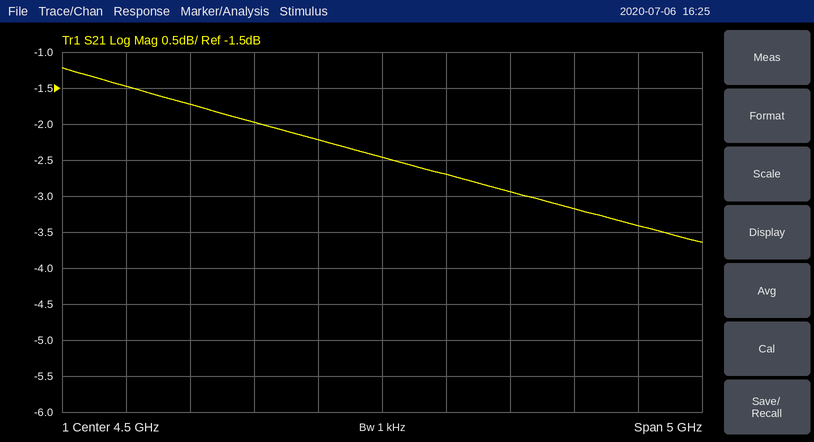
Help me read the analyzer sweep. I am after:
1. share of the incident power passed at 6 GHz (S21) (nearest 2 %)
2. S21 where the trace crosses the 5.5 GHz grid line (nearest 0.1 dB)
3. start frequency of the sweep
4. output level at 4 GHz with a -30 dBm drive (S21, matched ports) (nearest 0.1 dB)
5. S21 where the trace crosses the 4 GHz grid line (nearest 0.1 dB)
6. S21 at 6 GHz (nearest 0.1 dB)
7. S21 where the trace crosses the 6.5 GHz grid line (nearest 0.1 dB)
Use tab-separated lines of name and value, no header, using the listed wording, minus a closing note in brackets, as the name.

share of the incident power passed at 6 GHz (S21)	48 %
S21 where the trace crosses the 5.5 GHz grid line	-2.9 dB
start frequency of the sweep	2 GHz
output level at 4 GHz with a -30 dBm drive (S21, matched ports)	-32.2 dBm
S21 where the trace crosses the 4 GHz grid line	-2.2 dB
S21 at 6 GHz	-3.2 dB
S21 where the trace crosses the 6.5 GHz grid line	-3.4 dB
